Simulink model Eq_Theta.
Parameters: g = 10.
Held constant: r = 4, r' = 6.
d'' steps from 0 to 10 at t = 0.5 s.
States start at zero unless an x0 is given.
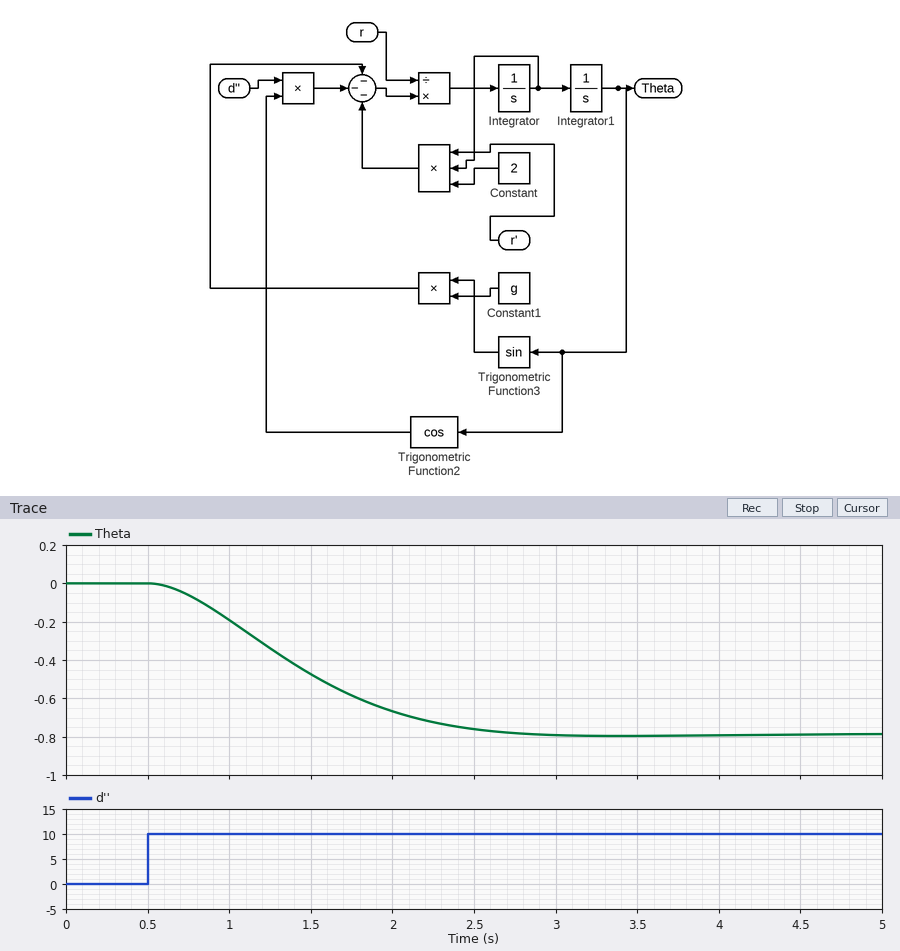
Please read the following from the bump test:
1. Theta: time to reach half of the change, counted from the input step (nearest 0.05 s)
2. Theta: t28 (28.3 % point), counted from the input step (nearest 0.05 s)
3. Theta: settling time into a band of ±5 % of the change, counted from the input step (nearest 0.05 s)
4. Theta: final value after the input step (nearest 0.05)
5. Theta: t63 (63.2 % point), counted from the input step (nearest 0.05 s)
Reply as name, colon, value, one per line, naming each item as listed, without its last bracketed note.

Theta: time to reach half of the change, counted from the input step: 0.85 s
Theta: t28 (28.3 % point), counted from the input step: 0.55 s
Theta: settling time into a band of ±5 % of the change, counted from the input step: 1.90 s
Theta: final value after the input step: -0.80
Theta: t63 (63.2 % point), counted from the input step: 1.05 s
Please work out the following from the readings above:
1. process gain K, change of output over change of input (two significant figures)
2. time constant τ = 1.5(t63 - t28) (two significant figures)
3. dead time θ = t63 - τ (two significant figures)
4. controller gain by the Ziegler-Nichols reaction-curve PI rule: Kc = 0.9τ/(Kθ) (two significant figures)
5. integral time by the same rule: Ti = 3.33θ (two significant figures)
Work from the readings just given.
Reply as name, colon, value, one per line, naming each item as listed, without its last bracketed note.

process gain K, change of output over change of input: -0.080
time constant τ = 1.5(t63 - t28): 0.75 s
dead time θ = t63 - τ: 0.30 s
controller gain by the Ziegler-Nichols reaction-curve PI rule: Kc = 0.9τ/(Kθ): -28
integral time by the same rule: Ti = 3.33θ: 1.00 s
